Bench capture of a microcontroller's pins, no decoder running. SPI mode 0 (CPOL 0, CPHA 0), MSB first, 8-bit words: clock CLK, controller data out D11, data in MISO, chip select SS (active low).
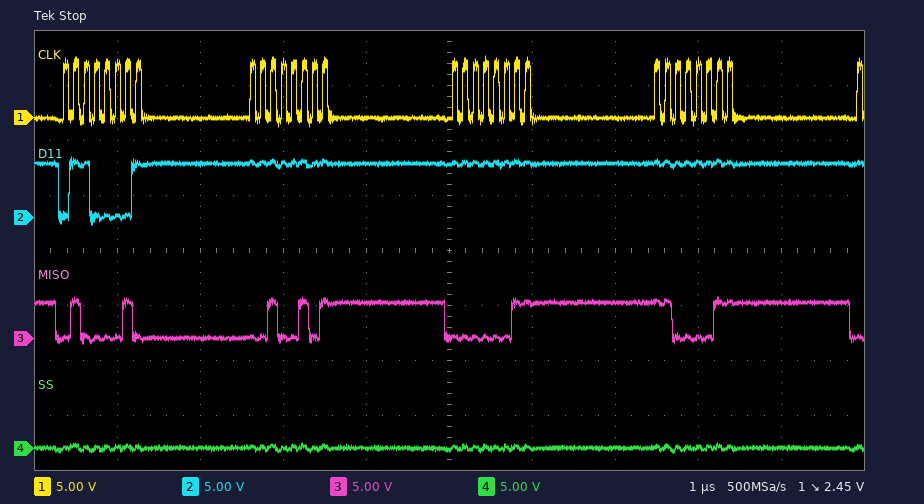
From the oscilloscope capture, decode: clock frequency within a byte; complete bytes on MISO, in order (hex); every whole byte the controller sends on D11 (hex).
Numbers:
8 MHz
0x42 0x25 0x03 0xC3
0x61 0xFF 0xFF 0xFF
